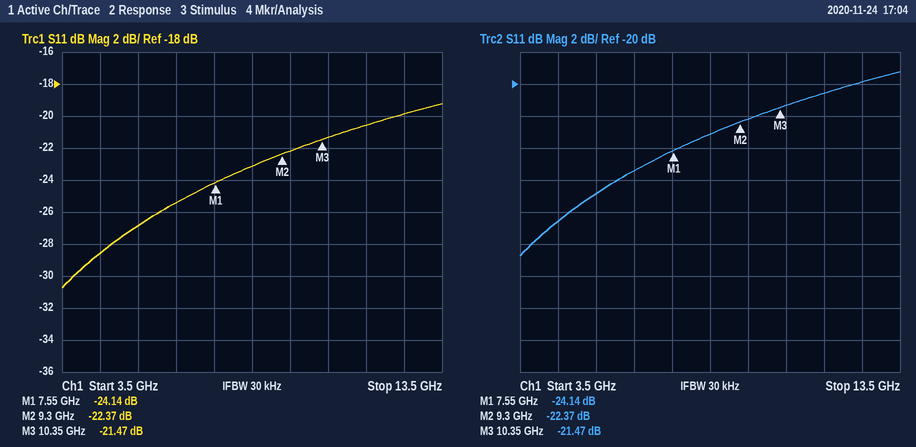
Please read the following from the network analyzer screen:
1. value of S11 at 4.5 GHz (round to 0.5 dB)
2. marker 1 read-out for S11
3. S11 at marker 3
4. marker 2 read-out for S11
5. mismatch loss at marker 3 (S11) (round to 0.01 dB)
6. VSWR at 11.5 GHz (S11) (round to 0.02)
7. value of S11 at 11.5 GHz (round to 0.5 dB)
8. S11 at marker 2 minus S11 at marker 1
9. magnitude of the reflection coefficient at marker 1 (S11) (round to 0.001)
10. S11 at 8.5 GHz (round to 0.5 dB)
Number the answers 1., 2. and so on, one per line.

1. -28.5 dB
2. -24.14 dB
3. -21.47 dB
4. -22.37 dB
5. 0.03 dB
6. 1.20
7. -20.5 dB
8. 1.77 dB
9. 0.062
10. -23.0 dB
